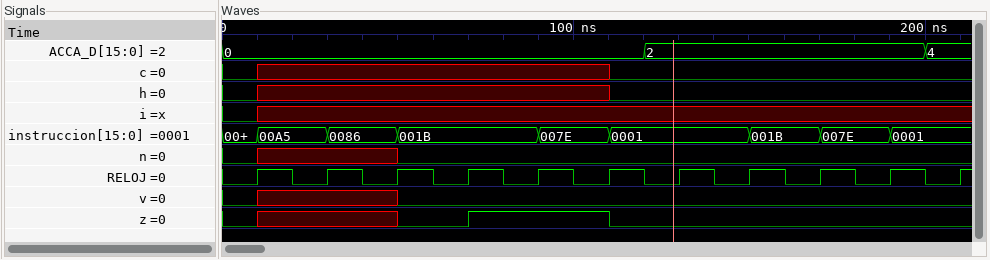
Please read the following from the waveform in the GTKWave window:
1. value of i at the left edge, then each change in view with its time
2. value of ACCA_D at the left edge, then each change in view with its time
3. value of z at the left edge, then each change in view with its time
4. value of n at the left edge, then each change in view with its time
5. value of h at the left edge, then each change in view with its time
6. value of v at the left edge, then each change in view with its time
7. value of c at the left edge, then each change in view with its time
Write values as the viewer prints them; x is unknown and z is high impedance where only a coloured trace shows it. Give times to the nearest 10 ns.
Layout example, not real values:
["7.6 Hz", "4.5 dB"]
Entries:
["0, x at 10 ns", "0, 2 at 120 ns, 4 at 200 ns", "0, x at 10 ns, 0 at 50 ns, 1 at 70 ns, 0 at 110 ns", "0, x at 10 ns, 0 at 50 ns", "0, x at 10 ns, 0 at 110 ns", "0, x at 10 ns, 0 at 50 ns", "0, x at 10 ns, 0 at 110 ns"]
